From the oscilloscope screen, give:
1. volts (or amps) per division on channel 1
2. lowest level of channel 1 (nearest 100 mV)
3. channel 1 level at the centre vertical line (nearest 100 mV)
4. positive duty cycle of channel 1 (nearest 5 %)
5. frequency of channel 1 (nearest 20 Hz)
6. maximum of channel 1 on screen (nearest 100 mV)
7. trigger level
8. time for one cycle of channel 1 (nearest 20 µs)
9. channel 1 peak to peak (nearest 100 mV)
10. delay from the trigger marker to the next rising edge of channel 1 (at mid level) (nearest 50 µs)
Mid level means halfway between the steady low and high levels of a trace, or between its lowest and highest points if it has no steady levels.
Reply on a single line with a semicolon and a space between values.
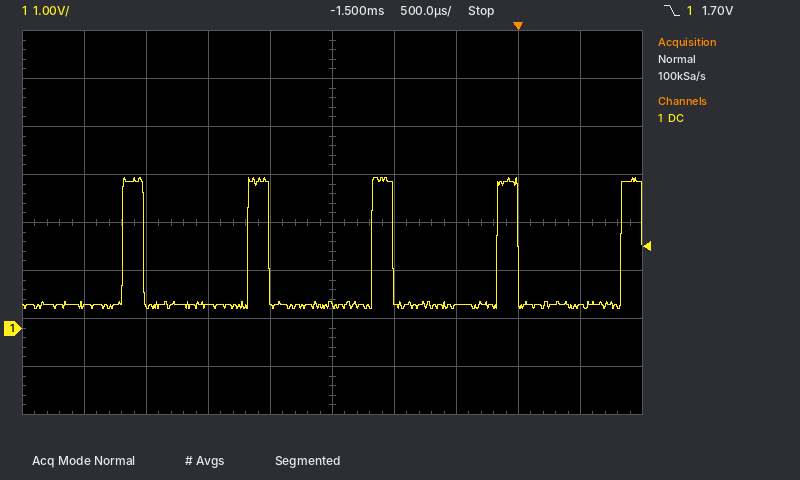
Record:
1 V; 400 mV; 500 mV; 15 %; 1.00 kHz; 3.1 V; 1.70 V; 1.00 ms; 2.7 V; 850 µs
